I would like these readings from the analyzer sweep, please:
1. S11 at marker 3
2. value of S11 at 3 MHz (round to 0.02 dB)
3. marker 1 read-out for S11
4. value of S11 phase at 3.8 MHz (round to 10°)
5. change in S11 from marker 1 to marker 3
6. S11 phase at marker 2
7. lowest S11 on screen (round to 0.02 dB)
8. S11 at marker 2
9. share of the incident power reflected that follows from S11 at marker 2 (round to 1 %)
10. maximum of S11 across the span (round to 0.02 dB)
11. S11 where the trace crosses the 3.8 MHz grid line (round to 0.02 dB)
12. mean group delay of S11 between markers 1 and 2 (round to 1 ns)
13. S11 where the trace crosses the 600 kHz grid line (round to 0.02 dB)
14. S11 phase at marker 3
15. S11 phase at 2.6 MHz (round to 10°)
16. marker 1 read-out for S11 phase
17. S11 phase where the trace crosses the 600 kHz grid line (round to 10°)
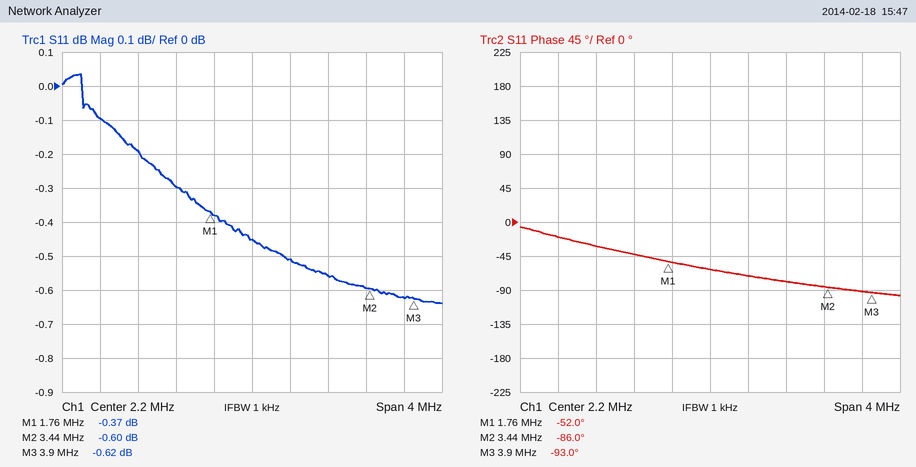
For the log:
-0.62 dB
-0.56 dB
-0.37 dB
-90°
-0.25 dB
-86.0°
-0.64 dB
-0.60 dB
87 %
0.04 dB
-0.62 dB
56 ns
-0.10 dB
-93.0°
-70°
-52.0°
-20°
